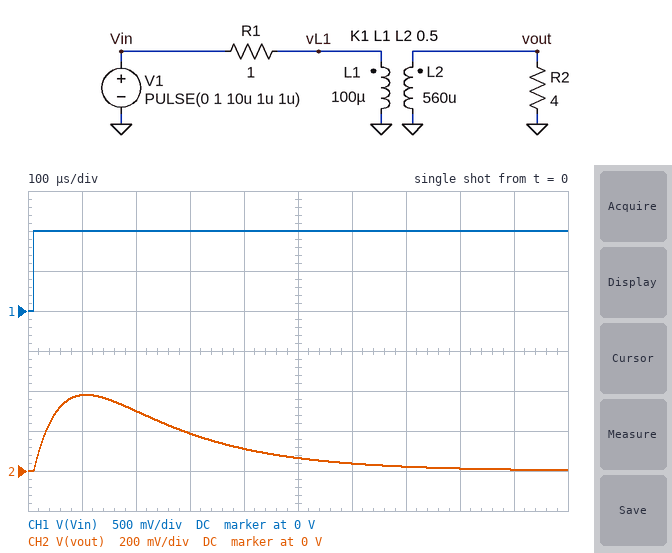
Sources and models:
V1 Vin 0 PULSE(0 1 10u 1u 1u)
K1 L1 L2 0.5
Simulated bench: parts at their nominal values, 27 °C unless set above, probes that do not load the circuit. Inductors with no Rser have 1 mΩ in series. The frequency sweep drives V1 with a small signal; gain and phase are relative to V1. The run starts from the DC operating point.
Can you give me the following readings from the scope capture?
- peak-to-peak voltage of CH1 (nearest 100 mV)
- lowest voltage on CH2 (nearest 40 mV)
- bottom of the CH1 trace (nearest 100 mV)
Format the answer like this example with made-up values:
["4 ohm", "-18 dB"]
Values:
["1.0 V", "0 V", "0 V"]
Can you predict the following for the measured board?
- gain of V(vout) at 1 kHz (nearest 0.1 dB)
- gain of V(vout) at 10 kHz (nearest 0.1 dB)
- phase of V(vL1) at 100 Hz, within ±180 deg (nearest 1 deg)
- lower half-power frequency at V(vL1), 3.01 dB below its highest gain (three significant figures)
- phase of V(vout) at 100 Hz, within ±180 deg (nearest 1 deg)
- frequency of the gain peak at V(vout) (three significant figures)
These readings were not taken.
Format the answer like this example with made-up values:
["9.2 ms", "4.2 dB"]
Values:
["-6.8 dB", "-15.3 dB", "84 deg", "2.23 kHz", "81 deg", "1.55 kHz"]
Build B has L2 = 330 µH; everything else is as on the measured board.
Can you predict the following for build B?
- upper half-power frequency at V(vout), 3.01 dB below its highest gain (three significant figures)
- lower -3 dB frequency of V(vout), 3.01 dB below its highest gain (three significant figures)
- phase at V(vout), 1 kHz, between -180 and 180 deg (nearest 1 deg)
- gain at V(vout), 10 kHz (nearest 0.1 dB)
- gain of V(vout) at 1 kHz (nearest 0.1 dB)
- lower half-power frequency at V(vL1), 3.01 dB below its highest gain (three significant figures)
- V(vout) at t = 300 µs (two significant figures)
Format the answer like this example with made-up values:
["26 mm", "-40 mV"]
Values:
["5.45 kHz", "752 Hz", "33 deg", "-13.2 dB", "-7.6 dB", "2.10 kHz", "120 mV"]
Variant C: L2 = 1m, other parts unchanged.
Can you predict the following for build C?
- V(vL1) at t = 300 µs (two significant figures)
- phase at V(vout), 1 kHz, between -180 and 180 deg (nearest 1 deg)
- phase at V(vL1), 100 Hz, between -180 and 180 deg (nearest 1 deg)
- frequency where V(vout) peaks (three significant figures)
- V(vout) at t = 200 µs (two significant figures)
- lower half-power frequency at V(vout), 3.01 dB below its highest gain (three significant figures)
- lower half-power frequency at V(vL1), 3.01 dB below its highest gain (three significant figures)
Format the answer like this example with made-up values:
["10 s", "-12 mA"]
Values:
["68 mV", "7 deg", "83 deg", "1.16 kHz", "330 mV", "401 Hz", "2.25 kHz"]
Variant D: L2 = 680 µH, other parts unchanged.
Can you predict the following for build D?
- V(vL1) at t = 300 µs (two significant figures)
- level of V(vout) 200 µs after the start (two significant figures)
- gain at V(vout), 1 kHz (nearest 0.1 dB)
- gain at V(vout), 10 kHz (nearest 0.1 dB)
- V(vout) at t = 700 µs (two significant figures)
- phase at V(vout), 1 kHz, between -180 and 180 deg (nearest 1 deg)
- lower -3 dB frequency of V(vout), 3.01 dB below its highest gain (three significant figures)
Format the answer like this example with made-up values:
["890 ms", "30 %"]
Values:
["73 mV", "320 mV", "-6.7 dB", "-16.1 dB", "32 mV", "16 deg", "512 Hz"]
